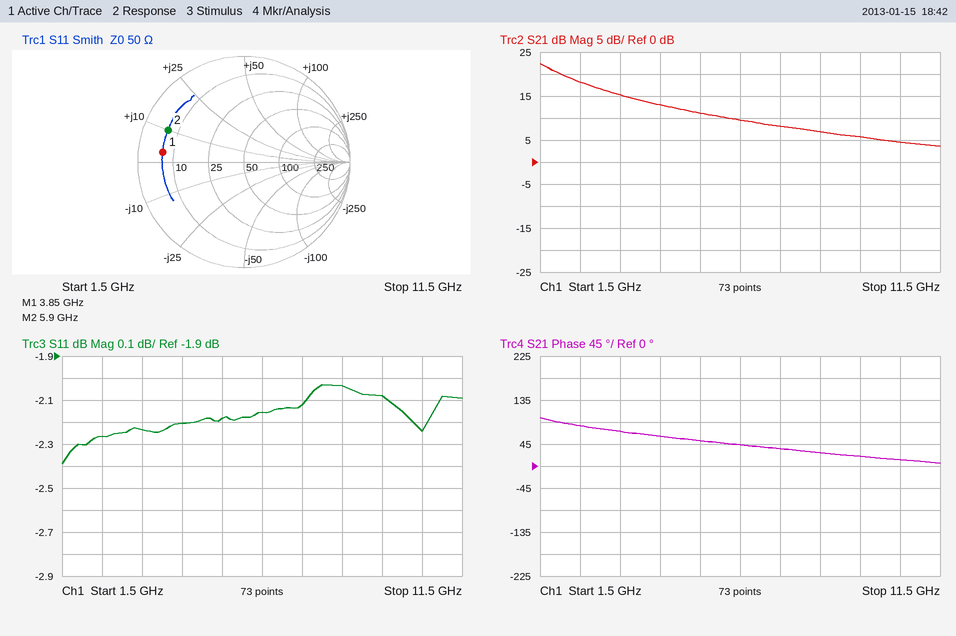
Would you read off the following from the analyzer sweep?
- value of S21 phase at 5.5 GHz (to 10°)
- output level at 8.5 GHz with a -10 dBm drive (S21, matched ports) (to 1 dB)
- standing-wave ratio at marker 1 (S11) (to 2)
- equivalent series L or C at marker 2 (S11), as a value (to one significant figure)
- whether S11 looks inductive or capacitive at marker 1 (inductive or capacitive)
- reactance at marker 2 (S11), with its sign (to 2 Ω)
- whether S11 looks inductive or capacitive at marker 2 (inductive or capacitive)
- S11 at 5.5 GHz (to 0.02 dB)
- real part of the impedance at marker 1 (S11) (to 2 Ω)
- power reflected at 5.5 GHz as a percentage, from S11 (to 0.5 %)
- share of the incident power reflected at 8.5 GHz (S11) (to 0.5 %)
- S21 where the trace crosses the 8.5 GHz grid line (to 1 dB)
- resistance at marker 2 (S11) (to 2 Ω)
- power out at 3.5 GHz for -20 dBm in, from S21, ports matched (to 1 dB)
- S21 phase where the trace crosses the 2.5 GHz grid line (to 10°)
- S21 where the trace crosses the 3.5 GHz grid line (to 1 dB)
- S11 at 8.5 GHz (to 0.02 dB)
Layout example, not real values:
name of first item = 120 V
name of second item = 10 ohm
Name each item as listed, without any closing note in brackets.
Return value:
value of S21 phase at 5.5 GHz = 50°
output level at 8.5 GHz with a -10 dBm drive (S21, matched ports) = -3 dBm
standing-wave ratio at marker 1 (S11) = 8
equivalent series L or C at marker 2 (S11), as a value = 300 pH
whether S11 looks inductive or capacitive at marker 1 = inductive
reactance at marker 2 (S11), with its sign = +10 Ω
whether S11 looks inductive or capacitive at marker 2 = inductive
S11 at 5.5 GHz = -2.18 dB
real part of the impedance at marker 1 (S11) = 6 Ω
power reflected at 5.5 GHz as a percentage, from S11 = 60.5 %
share of the incident power reflected at 8.5 GHz (S11) = 62.5 %
S21 where the trace crosses the 8.5 GHz grid line = 7 dB
resistance at marker 2 (S11) = 6 Ω
power out at 3.5 GHz for -20 dBm in, from S21, ports matched = -5 dBm
S21 phase where the trace crosses the 2.5 GHz grid line = 80°
S21 where the trace crosses the 3.5 GHz grid line = 15 dB
S11 at 8.5 GHz = -2.04 dB
